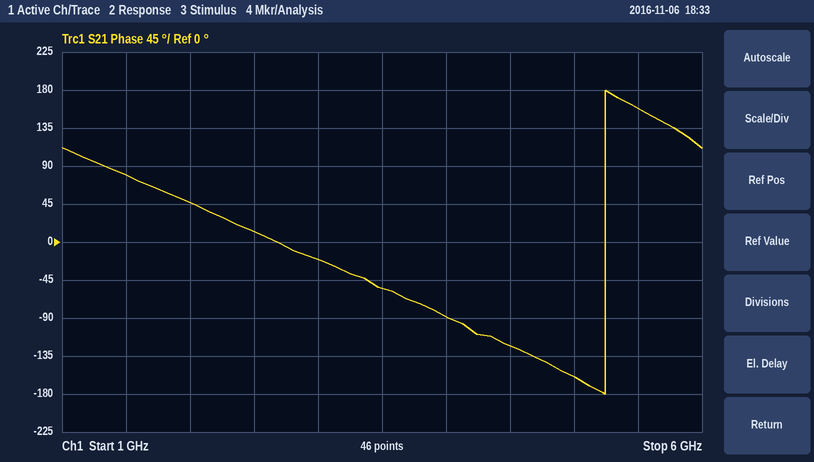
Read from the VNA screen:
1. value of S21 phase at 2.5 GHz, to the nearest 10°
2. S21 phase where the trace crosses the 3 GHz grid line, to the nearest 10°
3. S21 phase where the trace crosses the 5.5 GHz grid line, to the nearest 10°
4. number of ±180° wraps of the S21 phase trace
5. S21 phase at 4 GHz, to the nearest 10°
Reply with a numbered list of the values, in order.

1. 10°
2. -20°
3. 160°
4. 1
5. -90°
